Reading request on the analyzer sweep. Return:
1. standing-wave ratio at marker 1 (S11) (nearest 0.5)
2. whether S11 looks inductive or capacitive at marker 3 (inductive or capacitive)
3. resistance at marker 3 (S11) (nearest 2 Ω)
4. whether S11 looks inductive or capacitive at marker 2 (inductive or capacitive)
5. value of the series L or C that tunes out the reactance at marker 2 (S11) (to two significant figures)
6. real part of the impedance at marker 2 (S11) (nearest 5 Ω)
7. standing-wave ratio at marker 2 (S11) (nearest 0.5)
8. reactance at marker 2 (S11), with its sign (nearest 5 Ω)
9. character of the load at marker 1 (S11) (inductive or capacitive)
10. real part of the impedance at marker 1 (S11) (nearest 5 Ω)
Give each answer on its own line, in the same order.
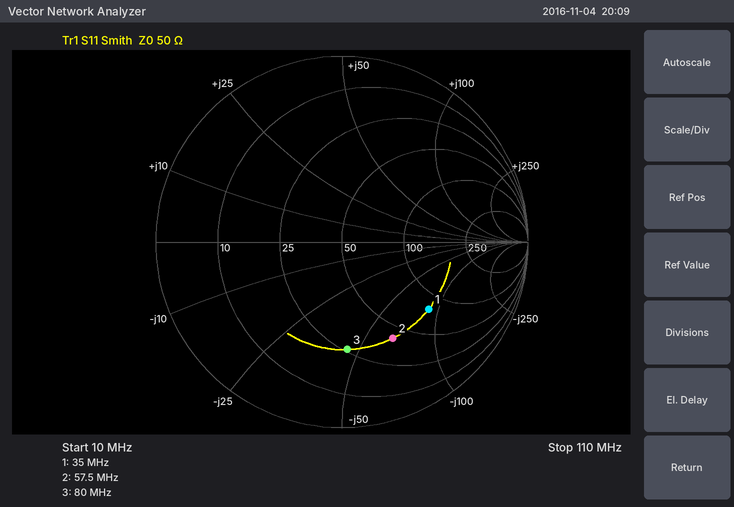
4.0
capacitive
26 Ω
capacitive
180 nH
40 Ω
4.0
-65 Ω
capacitive
80 Ω
